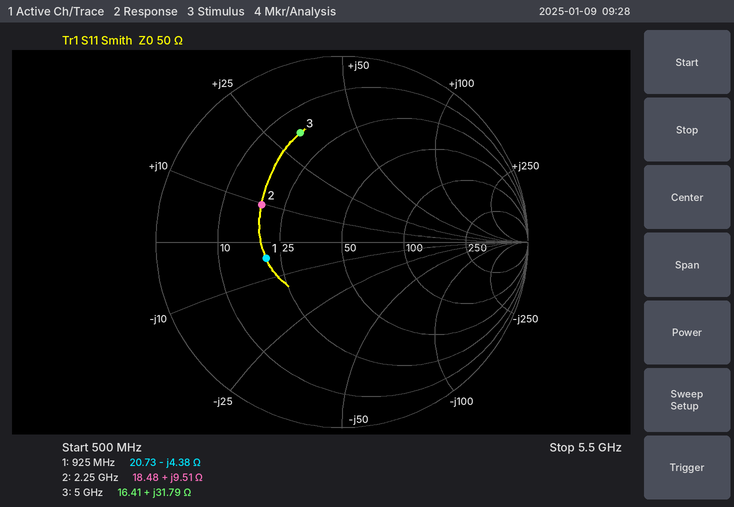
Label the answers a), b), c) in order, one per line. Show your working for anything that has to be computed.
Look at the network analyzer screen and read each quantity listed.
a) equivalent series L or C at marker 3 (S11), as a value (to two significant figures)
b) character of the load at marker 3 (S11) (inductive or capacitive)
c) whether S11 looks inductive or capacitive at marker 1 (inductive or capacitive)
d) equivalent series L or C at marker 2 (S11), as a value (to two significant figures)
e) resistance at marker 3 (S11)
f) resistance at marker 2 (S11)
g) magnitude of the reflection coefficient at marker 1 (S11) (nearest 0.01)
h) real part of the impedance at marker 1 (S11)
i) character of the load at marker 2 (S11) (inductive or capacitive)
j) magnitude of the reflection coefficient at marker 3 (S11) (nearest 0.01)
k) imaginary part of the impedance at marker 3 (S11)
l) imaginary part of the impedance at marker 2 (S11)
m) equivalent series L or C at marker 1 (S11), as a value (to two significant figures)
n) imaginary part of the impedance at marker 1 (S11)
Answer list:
a) L = 31.79 Ω/(2π × 5 GHz) ≈ 1.0 nH
b) inductive
c) capacitive
d) L = 9.51 Ω/(2π × 2.25 GHz) ≈ 673 pH, so 670 pH to two significant figures
e) 16.41 Ω
f) 18.48 Ω
g) 0.42
h) 20.73 Ω
i) inductive
j) 0.63
k) +31.79 Ω
l) +9.51 Ω
m) C = 1/(2π × 925 MHz × 4.38 Ω) ≈ 39 pF
n) -4.38 Ω
